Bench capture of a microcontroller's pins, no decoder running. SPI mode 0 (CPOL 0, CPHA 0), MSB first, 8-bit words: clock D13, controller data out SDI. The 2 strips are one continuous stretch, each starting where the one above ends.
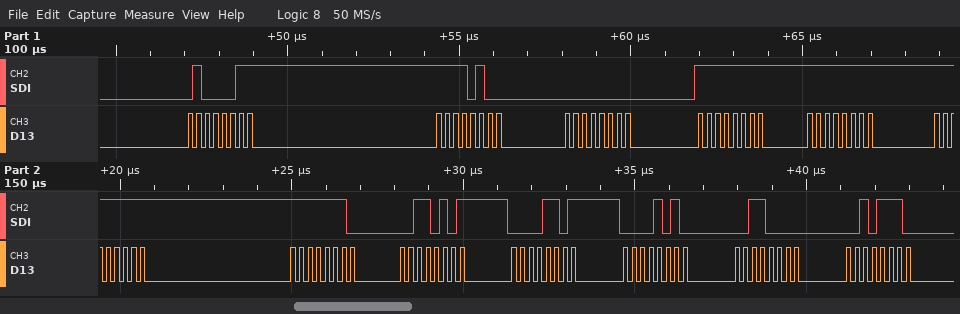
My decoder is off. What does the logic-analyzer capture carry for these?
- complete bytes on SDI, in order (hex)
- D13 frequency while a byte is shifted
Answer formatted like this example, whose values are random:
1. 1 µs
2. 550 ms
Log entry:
1. 43 F4 00 FF FF FF FE 35 0D 0A 30 2E
2. 4 MHz
